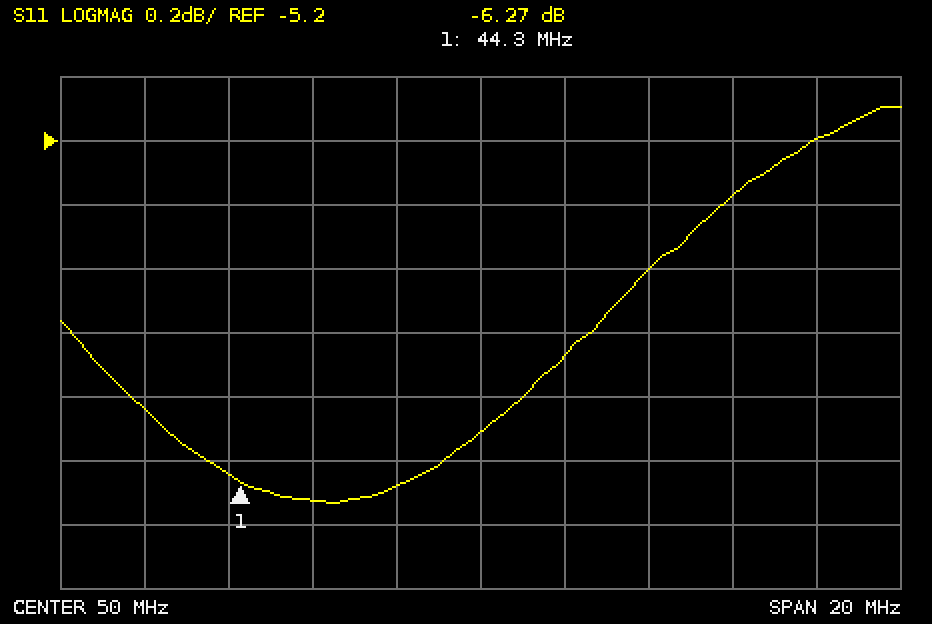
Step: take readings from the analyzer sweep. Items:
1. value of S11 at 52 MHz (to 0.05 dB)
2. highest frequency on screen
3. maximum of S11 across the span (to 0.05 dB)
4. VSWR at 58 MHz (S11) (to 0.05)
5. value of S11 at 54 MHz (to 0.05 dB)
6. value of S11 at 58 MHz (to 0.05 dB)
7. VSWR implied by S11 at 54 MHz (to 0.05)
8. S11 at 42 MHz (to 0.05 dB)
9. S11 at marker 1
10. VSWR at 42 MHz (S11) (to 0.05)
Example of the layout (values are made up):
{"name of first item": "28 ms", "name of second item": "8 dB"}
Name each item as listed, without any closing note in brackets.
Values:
{"value of S11 at 52 MHz": "-5.85 dB", "highest frequency on screen": "60 MHz", "maximum of S11 across the span": "-5.10 dB", "VSWR at 58 MHz (S11)": "3.45", "value of S11 at 54 MHz": "-5.60 dB", "value of S11 at 58 MHz": "-5.20 dB", "VSWR implied by S11 at 54 MHz": "3.20", "S11 at 42 MHz": "-6.05 dB", "S11 at marker 1": "-6.27 dB", "VSWR at 42 MHz (S11)": "3.00"}
